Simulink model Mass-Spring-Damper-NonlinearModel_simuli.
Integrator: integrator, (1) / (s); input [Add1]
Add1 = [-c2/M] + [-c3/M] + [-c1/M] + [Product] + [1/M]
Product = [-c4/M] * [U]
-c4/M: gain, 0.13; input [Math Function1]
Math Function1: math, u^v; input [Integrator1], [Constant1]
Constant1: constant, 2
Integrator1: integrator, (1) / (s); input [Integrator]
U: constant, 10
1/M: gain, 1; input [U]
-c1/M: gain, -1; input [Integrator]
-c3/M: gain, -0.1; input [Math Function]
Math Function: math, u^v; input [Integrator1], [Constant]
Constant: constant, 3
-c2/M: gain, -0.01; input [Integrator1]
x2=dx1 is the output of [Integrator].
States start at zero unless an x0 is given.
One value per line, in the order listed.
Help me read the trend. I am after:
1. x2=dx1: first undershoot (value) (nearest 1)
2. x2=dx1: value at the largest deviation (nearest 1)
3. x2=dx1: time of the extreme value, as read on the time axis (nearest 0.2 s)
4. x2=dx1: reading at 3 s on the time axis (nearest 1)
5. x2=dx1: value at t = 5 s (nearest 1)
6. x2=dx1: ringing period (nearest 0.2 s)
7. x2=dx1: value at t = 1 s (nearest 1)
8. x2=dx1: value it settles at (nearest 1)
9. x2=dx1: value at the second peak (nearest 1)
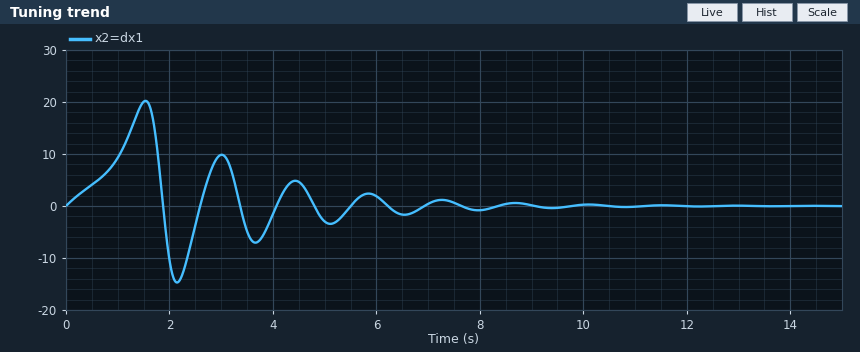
-15
20
1.6 s
10
-3
1.4 s
9
0
10
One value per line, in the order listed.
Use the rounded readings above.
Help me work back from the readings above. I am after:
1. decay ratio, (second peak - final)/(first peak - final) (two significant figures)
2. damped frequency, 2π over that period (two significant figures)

0.50
4.5 rad/s
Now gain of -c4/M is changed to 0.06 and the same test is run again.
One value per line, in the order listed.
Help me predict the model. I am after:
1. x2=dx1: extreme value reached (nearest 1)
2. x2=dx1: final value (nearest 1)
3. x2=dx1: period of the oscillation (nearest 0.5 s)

8
0
2.0 s
